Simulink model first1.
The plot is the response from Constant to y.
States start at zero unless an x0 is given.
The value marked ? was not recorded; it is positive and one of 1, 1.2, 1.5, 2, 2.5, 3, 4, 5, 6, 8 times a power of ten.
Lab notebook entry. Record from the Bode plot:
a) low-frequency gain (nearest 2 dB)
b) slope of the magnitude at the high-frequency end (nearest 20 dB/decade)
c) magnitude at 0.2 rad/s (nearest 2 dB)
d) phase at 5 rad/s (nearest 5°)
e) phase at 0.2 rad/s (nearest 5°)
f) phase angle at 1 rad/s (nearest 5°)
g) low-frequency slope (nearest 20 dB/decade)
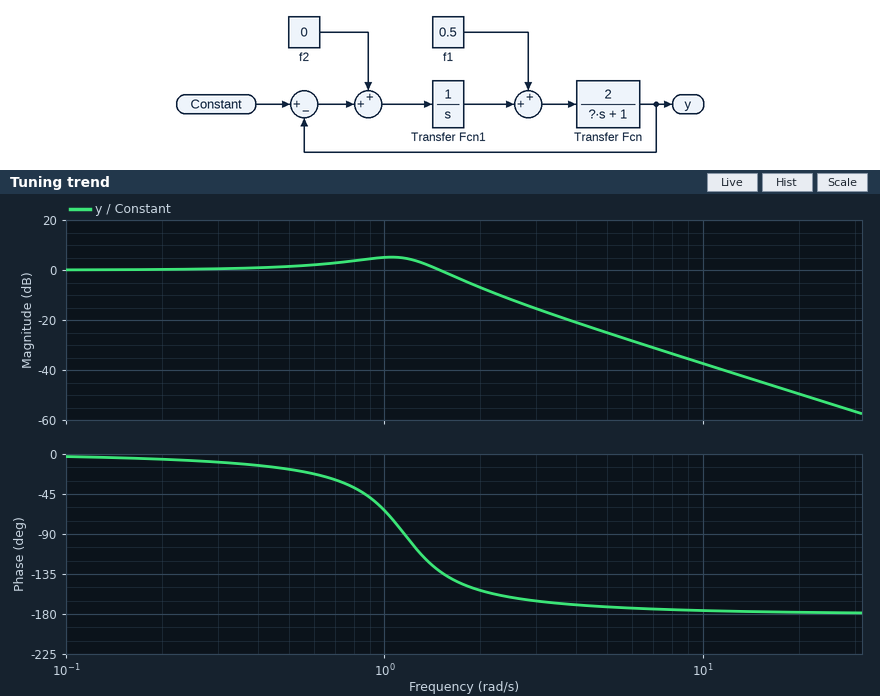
0 dB
-40 dB/decade
0 dB
-170°
-5°
-65°
0 dB/decade
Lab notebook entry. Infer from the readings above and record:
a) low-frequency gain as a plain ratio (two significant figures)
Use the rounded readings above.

1.0
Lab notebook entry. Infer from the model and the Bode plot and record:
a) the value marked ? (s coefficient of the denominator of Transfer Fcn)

1.5
